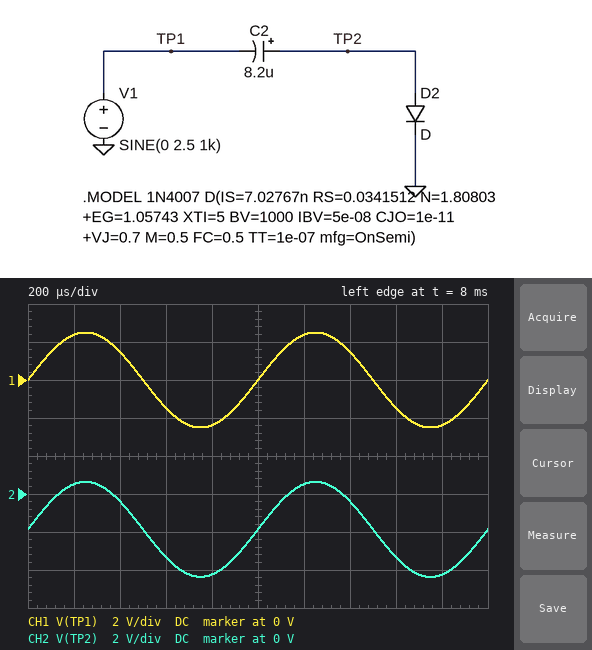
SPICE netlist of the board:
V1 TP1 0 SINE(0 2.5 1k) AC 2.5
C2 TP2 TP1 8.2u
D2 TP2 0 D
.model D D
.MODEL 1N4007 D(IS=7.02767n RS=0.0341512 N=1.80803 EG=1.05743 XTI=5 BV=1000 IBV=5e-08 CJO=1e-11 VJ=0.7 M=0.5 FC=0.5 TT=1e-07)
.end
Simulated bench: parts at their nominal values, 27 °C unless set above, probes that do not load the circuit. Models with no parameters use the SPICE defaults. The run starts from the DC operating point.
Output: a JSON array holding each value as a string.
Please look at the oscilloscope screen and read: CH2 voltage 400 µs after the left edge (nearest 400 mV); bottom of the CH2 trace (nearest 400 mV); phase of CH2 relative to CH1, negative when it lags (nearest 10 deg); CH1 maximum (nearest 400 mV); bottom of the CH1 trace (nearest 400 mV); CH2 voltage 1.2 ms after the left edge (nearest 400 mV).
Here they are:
["-400 mV", "-4.4 V", "0 deg", "2.4 V", "-2.4 V", "400 mV"]
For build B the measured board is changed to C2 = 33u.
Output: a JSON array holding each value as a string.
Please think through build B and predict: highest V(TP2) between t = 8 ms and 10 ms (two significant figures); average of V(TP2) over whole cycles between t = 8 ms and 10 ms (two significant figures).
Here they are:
["680 mV", "-1.8 V"]
